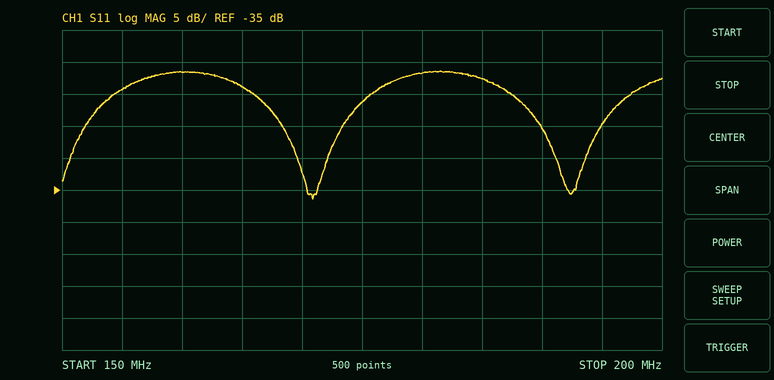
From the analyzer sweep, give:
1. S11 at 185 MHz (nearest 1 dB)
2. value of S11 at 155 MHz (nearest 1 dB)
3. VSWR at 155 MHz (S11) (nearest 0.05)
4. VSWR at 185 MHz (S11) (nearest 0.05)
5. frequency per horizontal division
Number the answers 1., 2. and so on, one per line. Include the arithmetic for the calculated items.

1. -18 dB
2. -19 dB
3. |Γ| = 10^(-19/20) = 0.1122; VSWR = (1 + 0.1122)/(1 − 0.1122) ≈ 1.25
4. |Γ| = 10^(-18/20) = 0.1259; VSWR = (1 + 0.1259)/(1 − 0.1259) ≈ 1.29, so 1.30 to the nearest 0.05
5. 5 MHz
